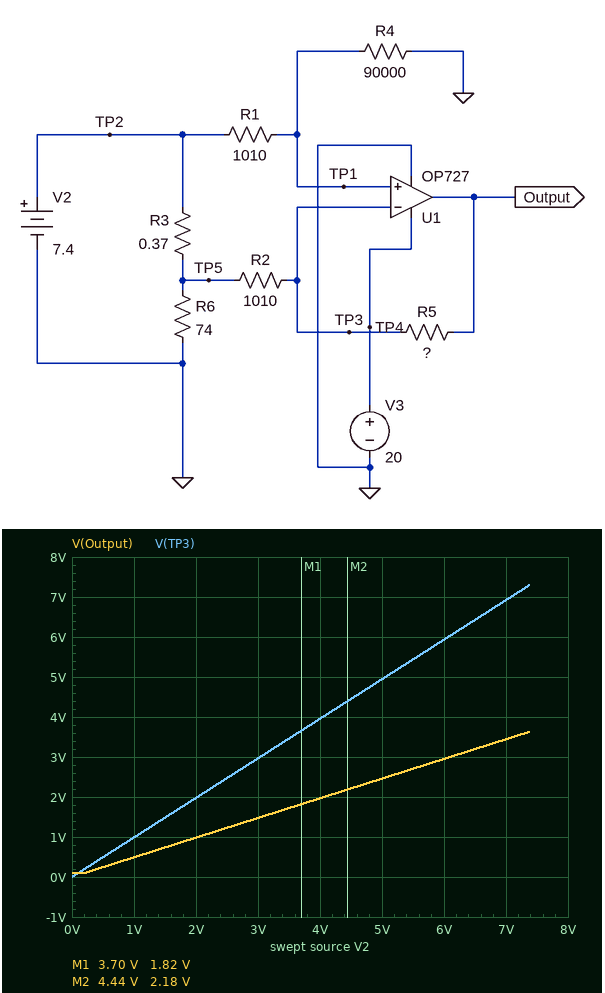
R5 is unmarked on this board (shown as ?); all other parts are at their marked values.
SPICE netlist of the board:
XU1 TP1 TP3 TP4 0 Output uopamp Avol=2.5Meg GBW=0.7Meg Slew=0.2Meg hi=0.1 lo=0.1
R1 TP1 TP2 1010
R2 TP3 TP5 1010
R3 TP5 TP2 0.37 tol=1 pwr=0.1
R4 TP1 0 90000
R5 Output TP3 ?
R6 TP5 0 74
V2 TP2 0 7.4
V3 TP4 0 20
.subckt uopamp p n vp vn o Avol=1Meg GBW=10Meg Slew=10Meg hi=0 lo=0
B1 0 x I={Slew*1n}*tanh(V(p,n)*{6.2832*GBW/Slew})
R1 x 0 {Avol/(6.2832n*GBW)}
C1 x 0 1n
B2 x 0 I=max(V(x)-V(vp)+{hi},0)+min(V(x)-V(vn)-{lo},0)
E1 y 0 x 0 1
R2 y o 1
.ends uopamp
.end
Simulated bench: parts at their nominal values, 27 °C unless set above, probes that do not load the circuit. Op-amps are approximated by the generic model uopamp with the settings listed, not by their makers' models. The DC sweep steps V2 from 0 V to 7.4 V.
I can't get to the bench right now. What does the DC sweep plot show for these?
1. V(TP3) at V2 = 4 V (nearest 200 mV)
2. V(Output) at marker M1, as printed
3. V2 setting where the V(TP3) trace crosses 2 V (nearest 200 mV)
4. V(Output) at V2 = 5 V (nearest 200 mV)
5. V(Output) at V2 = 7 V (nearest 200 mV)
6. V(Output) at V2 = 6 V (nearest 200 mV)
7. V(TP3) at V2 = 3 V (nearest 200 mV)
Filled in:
4.0 V
1.82 V
2.0 V
2.4 V
3.4 V
3.0 V
3.0 V
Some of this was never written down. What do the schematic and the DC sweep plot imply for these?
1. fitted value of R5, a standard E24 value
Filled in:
82 kΩ
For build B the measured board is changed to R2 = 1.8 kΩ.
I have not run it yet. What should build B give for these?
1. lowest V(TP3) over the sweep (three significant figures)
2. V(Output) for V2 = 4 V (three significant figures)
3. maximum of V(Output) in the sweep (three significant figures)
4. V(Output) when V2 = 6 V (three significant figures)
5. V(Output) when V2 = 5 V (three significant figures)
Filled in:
2.15 mV
2.84 V
5.25 V
4.26 V
3.55 V
